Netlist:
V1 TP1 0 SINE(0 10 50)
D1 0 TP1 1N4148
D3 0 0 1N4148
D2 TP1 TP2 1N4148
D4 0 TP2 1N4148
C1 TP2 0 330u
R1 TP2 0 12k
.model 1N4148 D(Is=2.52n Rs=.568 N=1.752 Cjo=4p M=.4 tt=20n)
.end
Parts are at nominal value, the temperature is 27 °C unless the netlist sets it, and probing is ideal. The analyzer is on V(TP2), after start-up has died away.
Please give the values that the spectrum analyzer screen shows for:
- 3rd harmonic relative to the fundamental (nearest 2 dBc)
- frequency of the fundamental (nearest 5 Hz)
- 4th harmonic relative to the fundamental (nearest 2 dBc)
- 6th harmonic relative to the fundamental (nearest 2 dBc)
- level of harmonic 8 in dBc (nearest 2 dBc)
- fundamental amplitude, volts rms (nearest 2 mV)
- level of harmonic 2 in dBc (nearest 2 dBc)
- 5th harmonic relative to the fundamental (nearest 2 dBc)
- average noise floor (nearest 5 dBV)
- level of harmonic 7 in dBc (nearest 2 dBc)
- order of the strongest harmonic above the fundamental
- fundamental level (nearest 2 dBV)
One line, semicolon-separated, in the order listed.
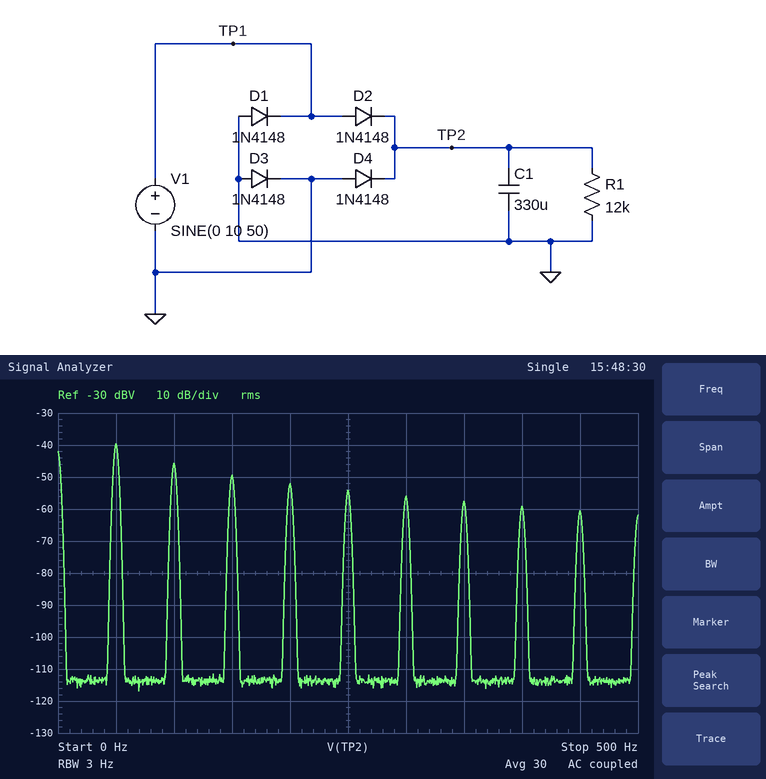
-10 dBc; 50 Hz; -12 dBc; -16 dBc; -20 dBc; 10 mV; -6 dBc; -14 dBc; -115 dBV; -18 dBc; 2; -40 dBV
